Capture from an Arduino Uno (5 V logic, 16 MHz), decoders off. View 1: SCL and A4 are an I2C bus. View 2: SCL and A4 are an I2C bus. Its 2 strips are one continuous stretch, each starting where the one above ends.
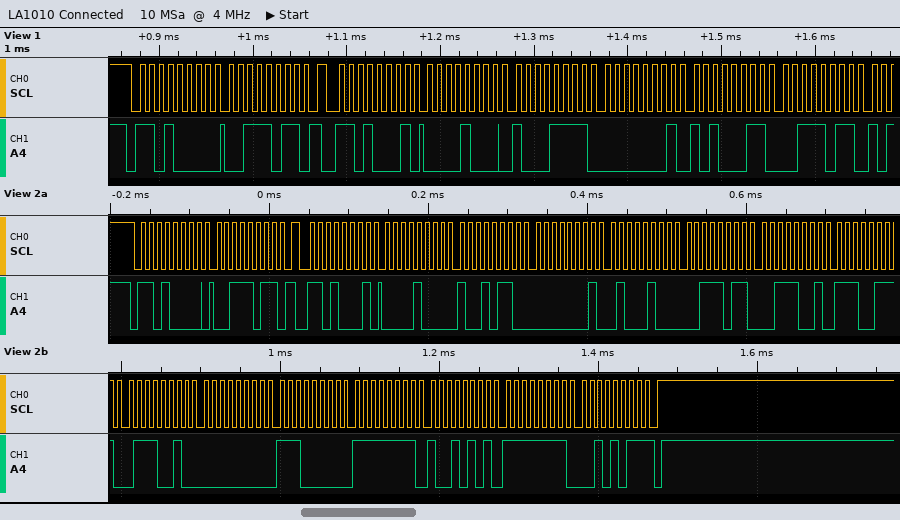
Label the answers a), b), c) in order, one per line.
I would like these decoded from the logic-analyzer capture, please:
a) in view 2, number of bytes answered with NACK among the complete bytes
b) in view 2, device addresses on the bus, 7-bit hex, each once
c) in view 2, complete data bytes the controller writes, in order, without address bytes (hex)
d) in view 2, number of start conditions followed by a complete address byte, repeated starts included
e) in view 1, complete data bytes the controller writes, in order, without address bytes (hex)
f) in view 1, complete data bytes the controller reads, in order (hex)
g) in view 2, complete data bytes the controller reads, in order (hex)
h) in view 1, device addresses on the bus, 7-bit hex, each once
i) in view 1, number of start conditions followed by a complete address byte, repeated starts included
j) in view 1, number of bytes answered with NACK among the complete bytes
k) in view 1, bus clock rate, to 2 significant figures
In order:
a) 1
b) 0x68
c) 3B
d) 2
e) 3B
f) 08 8F 01 A3 3B
g) 08 96 01 44 3B 39 E7 72 00 E0 FF 95 FF 2B
h) 0x68
i) 2
j) 0
k) 100 kHz
